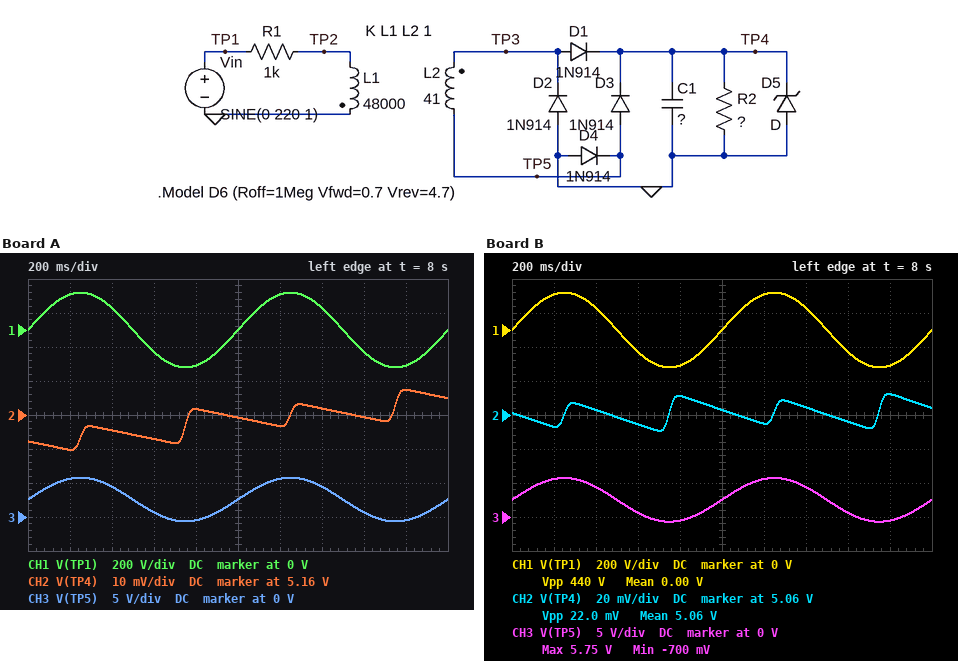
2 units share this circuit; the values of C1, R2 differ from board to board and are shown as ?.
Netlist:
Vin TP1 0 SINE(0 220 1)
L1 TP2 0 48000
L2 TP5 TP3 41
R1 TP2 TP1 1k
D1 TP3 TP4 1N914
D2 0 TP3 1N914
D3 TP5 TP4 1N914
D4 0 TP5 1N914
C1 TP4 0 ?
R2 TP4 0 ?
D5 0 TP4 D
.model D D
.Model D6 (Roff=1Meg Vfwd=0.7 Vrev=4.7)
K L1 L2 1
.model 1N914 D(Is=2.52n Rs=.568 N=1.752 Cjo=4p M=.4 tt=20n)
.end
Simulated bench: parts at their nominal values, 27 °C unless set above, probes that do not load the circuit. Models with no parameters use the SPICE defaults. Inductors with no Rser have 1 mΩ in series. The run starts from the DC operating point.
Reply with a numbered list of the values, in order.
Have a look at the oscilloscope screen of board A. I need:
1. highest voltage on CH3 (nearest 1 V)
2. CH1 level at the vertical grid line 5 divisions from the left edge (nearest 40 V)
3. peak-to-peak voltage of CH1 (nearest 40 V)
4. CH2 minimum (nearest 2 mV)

1. 6 V
2. 0 V
3. 440 V
4. 5.150 V
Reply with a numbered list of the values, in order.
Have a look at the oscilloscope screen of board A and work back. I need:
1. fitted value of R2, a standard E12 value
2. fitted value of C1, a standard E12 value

1. 27 kΩ
2. 15 mF
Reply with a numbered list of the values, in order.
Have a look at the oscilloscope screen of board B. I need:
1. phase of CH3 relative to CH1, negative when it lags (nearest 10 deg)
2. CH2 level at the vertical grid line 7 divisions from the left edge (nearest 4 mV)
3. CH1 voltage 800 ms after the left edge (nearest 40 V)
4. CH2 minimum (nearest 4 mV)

1. 0 deg
2. 5.064 V
3. -200 V
4. 5.052 V
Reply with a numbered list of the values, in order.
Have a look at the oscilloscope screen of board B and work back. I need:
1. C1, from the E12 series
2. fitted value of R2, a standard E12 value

1. 18 mF
2. 6.8 kΩ
